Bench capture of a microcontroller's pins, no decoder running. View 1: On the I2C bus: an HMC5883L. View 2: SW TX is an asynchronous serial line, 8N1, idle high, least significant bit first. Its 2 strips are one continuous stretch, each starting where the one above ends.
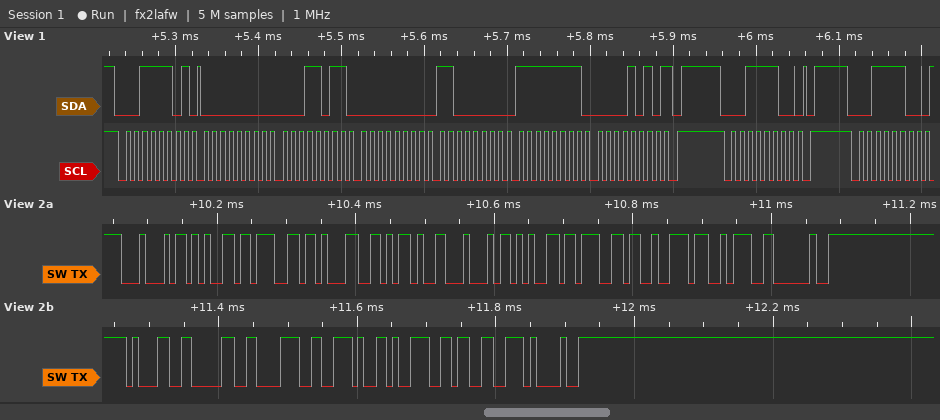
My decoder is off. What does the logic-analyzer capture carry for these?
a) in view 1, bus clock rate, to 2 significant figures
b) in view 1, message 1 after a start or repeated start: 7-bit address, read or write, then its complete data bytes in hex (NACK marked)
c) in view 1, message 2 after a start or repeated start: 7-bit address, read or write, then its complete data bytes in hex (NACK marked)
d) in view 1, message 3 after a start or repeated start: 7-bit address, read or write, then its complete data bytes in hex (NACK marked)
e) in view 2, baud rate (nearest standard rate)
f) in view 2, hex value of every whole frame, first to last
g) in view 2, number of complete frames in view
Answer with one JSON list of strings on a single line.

["100 kHz", "0x1E read: 00 1B 00 C0 FF 0A NACK", "0x1E write", "0x1E write", "115200 baud", "0x44 0x65 0x67 0x31 0x2D 0x44 0x65 0x67 0x72 0x3A 0x20 0x31 0x30 0x38 0x2E 0x39 0x33 0x21", "18"]
